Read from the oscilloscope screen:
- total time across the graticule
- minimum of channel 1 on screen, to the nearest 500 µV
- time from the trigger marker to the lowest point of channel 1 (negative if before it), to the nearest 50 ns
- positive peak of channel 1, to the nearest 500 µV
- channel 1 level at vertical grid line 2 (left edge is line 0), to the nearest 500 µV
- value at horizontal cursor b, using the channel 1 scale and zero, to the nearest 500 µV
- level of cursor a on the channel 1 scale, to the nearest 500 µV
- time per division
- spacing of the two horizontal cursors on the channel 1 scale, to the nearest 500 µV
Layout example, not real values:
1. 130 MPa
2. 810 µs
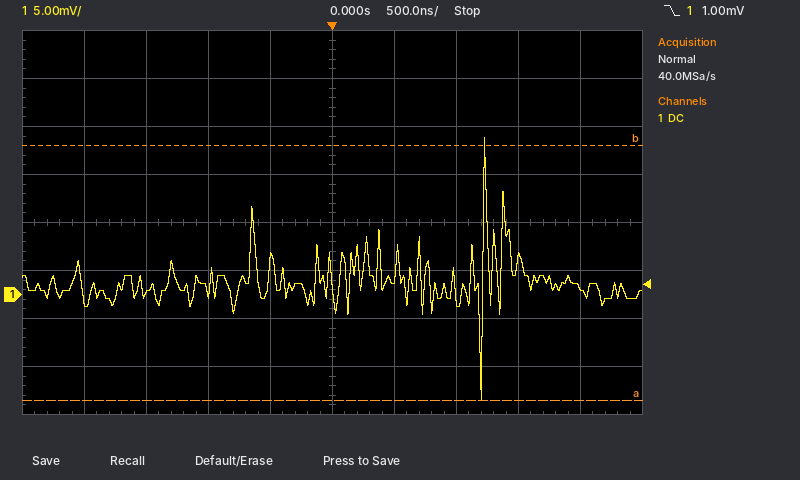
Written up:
1. 5 µs
2. -11.0 mV
3. +1.20 µs
4. 16.5 mV
5. 0.0 mV
6. 15.5 mV
7. -11.0 mV
8. 500 ns
9. 26.5 mV
